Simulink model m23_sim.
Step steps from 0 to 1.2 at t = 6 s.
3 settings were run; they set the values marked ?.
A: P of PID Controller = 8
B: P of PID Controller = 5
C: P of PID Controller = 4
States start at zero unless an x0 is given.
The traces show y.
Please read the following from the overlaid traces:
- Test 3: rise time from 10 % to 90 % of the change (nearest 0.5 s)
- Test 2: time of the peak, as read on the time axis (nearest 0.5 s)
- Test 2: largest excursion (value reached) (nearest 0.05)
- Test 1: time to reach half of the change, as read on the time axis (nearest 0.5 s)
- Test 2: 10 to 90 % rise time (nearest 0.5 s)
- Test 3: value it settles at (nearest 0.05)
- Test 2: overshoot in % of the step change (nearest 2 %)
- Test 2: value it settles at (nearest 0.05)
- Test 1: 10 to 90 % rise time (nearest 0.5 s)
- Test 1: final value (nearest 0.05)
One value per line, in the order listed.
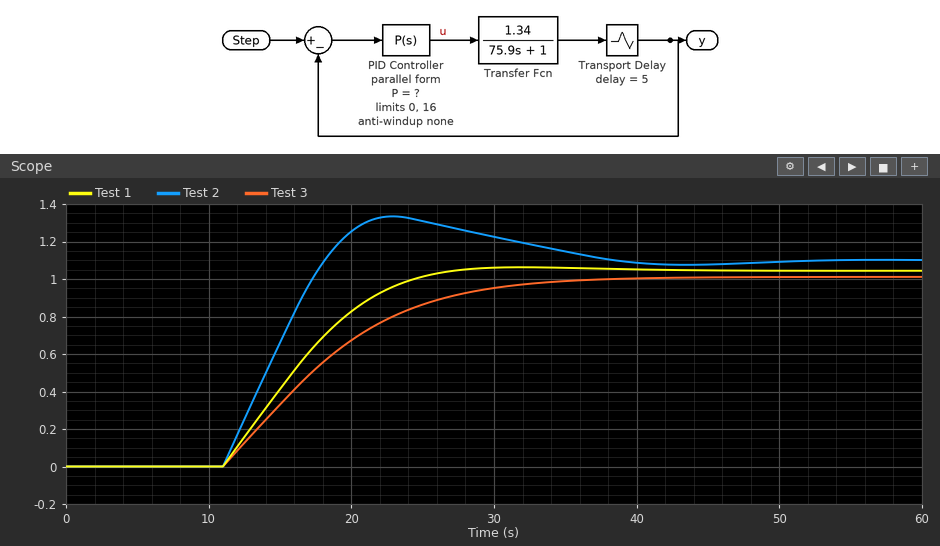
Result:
15.0 s
23.0 s
1.35
16.0 s
5.5 s
1.00
22 %
1.10
10.5 s
1.05
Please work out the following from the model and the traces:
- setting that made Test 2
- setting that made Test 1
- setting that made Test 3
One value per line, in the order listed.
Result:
A
B
C
